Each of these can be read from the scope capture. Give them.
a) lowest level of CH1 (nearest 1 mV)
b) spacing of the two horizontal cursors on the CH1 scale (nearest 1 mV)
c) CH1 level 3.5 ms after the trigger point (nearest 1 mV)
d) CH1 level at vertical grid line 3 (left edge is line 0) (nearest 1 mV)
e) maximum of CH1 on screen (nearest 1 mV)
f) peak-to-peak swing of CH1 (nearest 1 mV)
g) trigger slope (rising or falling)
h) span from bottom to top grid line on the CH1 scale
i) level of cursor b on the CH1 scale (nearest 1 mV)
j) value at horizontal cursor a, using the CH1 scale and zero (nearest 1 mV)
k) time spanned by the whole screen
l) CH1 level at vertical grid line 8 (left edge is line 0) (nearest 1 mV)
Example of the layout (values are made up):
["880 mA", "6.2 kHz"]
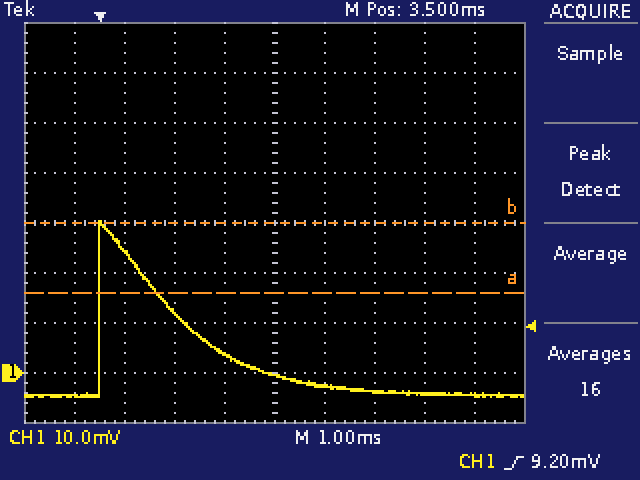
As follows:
["-5 mV", "14 mV", "0 mV", "12 mV", "30 mV", "35 mV", "rising", "80 mV", "30 mV", "16 mV", "10 ms", "-4 mV"]
